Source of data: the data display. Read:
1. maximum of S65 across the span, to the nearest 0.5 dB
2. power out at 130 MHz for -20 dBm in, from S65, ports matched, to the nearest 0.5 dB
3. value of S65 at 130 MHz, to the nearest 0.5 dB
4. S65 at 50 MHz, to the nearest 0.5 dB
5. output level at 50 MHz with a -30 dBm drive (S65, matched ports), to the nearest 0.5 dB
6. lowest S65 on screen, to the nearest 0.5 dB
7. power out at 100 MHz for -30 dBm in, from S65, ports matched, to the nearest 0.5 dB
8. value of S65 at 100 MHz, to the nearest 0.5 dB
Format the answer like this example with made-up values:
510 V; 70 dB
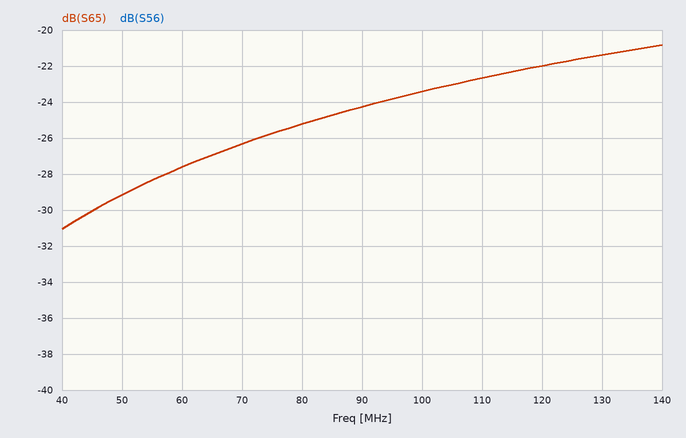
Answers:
-21.0 dB; -41.5 dBm; -21.5 dB; -29.0 dB; -59.0 dBm; -31.0 dB; -53.5 dBm; -23.5 dB
